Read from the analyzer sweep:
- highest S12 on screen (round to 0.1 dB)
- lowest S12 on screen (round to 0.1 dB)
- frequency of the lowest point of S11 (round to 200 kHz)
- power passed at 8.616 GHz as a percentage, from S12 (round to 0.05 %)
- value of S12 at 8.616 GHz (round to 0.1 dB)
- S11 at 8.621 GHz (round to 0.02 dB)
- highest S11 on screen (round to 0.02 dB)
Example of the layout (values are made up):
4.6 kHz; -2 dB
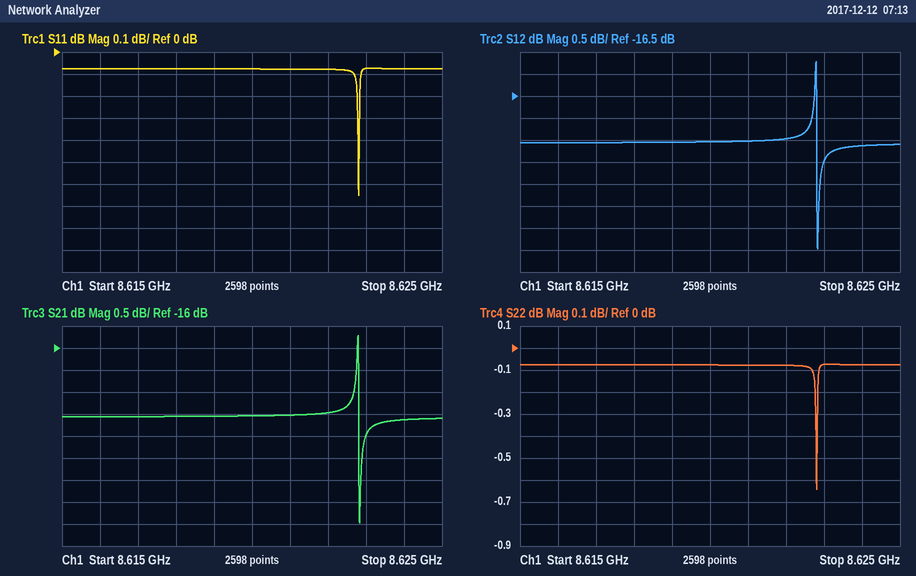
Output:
-15.7 dB; -20.0 dB; 8.6228 GHz; 1.75 %; -17.6 dB; -0.08 dB; -0.08 dB
